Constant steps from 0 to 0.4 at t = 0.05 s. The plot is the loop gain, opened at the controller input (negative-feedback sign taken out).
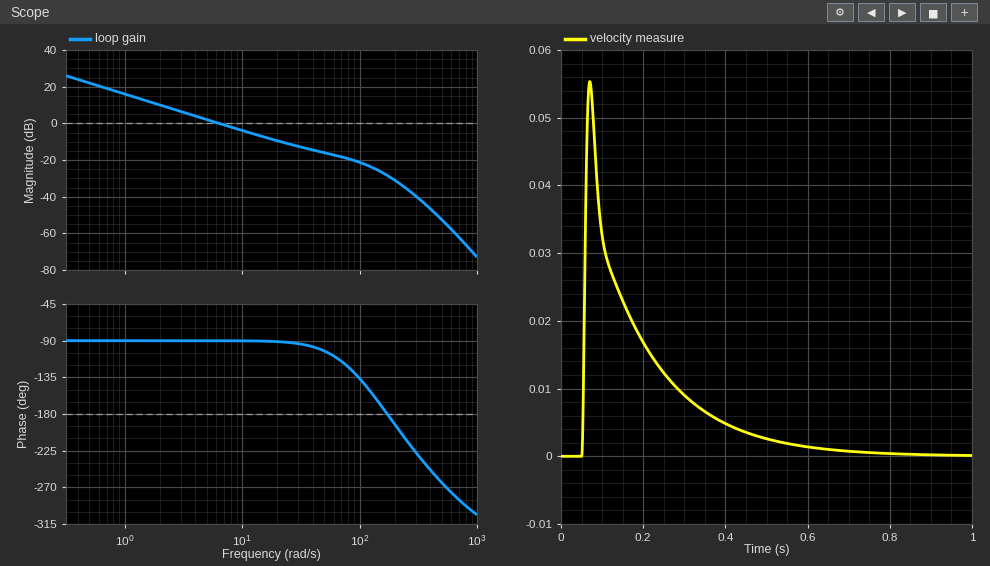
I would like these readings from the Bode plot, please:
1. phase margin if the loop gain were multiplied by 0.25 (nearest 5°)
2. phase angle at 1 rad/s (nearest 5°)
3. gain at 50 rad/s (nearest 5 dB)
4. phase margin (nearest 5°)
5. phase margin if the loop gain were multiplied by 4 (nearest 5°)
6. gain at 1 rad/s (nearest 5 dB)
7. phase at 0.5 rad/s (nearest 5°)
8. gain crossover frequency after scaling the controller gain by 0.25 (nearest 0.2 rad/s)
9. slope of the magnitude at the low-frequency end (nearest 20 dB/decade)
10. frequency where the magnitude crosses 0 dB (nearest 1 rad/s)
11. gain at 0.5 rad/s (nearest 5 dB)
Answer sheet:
90°
-90°
-15 dB
90°
85°
15 dB
-90°
1.6 rad/s
-20 dB/decade
6 rad/s
20 dB
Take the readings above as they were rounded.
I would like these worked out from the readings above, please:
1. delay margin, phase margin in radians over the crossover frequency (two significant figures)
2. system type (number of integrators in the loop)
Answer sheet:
0.26 s
1
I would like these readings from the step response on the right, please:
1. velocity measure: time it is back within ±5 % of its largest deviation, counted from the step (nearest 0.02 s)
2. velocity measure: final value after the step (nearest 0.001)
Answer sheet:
0.44 s
0.000
